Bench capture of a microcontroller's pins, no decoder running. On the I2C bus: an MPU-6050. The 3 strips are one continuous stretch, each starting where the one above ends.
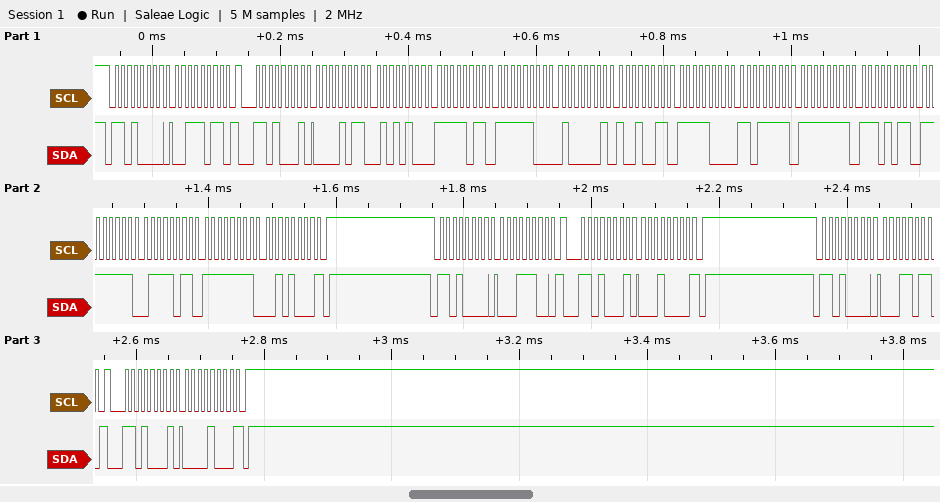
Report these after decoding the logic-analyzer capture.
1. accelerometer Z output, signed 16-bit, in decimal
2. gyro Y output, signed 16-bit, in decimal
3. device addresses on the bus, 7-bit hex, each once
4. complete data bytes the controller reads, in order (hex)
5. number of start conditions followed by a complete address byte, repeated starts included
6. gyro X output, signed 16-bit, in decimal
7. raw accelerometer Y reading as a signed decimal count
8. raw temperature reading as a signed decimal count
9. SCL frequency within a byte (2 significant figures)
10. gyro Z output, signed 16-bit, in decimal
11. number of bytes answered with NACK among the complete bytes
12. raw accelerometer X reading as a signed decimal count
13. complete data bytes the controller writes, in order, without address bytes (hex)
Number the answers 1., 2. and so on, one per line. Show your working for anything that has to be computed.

1. 0x4193 = 16787
2. 0xFF7B = -133
3. 0x68
4. 0B 54 FB FC 41 93 F8 DF FF EB FF 7B FF 28 10 08
5. 6
6. 0xFFEB = -21
7. 0xFBFC = -1028
8. 0xF8DF = -1825
9. 100 kHz
10. 0xFF28 = -216
11. 3
12. 0x0B54 = 2900
13. 3B 1C 1B
